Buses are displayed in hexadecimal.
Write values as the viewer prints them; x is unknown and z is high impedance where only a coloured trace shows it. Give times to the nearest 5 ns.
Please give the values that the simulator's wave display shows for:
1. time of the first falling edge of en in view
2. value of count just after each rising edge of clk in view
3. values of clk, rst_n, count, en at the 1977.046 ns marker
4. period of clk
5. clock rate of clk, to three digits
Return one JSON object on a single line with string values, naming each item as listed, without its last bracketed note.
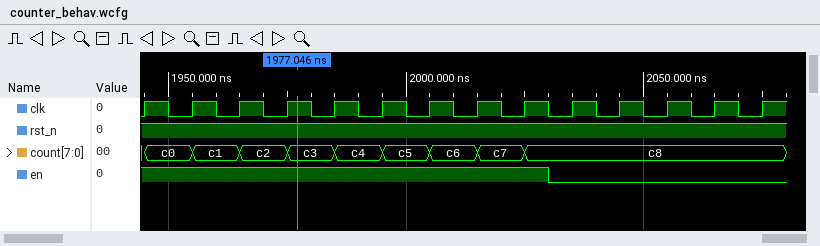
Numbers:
{"time of the first falling edge of en in view": "2030 ns", "value of count just after each rising edge of clk in view": "c0, c1, c2, c3, c4, c5, c6, c7, c8, c8, c8, c8, c8, c8", "values of clk, rst_n, count, en at the 1977.046 ns marker": "clk=1, rst_n=1, count=c3, en=1", "period of clk": "10 ns", "clock rate of clk, to three digits": "100 MHz"}
